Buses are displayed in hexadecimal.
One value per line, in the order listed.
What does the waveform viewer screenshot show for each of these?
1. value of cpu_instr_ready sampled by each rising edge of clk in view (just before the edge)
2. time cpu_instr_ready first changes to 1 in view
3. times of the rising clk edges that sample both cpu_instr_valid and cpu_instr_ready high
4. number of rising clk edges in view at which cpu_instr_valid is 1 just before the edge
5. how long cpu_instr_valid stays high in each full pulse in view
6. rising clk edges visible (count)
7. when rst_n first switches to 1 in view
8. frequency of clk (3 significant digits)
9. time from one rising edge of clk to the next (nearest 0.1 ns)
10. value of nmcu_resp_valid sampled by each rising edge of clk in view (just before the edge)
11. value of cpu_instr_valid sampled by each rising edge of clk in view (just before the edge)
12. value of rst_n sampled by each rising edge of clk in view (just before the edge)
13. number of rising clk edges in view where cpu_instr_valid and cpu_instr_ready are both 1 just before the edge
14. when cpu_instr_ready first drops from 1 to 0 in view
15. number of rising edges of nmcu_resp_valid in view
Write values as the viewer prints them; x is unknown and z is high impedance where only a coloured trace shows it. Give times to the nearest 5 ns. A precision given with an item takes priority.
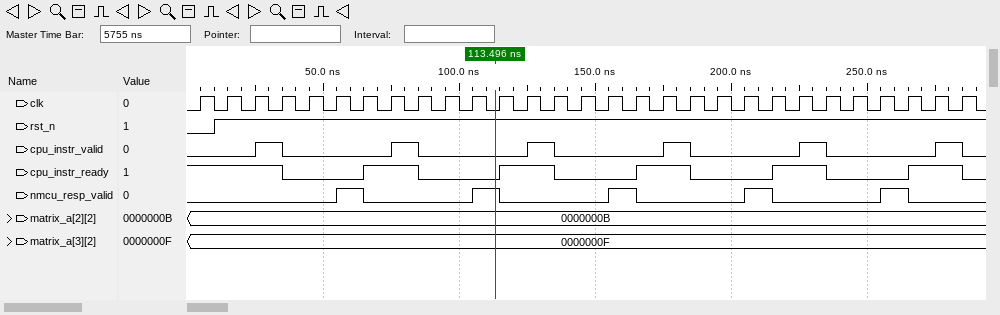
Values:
1 1 1 1 0 0 0 1 1 0 0 0 1 1 0 0 0 1 1 0 0 0 1 1 0 0 0 1 1
65 ns
35 ns, 85 ns, 135 ns, 185 ns, 235 ns, 285 ns
6
10 ns, 10 ns, 10 ns, 10 ns, 10 ns, 10 ns
29
10 ns
100 MHz
10 ns
0 0 0 0 0 0 1 0 0 0 0 1 0 0 0 0 1 0 0 0 0 1 0 0 0 0 1 0 0
0 0 0 1 0 0 0 0 1 0 0 0 0 1 0 0 0 0 1 0 0 0 0 1 0 0 0 0 1
0 1 1 1 1 1 1 1 1 1 1 1 1 1 1 1 1 1 1 1 1 1 1 1 1 1 1 1 1
6
35 ns
5
